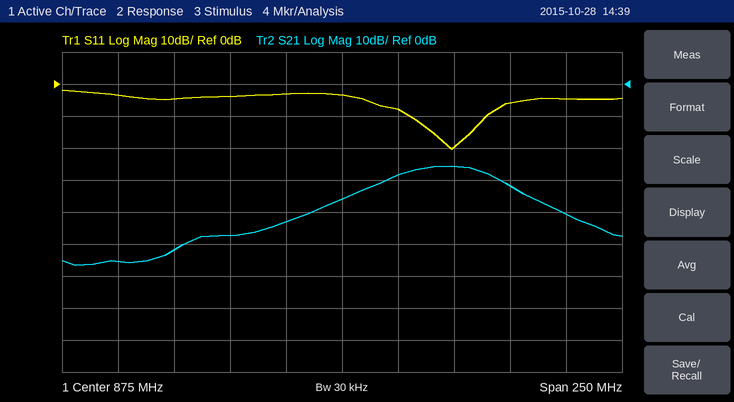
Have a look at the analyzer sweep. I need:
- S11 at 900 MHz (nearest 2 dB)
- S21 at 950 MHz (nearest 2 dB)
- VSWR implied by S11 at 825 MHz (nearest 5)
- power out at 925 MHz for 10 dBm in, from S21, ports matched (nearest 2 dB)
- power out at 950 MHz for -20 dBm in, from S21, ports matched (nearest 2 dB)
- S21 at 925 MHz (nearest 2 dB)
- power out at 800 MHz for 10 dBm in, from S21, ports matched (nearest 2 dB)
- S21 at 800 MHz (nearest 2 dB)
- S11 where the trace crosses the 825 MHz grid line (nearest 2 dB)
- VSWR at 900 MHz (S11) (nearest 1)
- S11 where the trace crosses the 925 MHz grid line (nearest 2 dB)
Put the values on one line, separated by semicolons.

-8 dB; -32 dB; 5; -16 dBm; -52 dBm; -26 dB; -42 dBm; -52 dB; -4 dB; 2; -20 dB
